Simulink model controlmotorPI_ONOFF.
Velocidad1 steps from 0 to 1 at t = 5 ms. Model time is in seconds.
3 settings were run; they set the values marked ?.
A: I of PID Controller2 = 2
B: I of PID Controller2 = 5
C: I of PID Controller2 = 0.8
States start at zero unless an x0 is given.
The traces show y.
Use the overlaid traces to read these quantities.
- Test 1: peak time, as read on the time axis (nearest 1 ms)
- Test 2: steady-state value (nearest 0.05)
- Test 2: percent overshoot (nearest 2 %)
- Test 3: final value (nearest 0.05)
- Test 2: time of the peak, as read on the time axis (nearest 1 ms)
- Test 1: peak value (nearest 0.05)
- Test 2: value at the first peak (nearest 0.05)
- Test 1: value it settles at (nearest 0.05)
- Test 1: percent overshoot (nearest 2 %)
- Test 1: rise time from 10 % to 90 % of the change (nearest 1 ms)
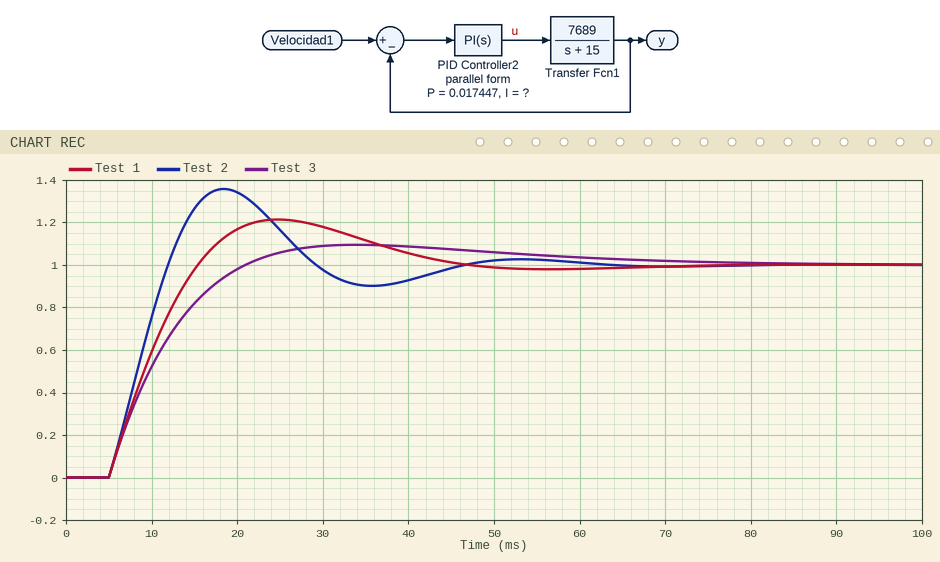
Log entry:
25 ms
1.00
36 %
1.00
18 ms
1.20
1.35
1.00
22 %
8 ms
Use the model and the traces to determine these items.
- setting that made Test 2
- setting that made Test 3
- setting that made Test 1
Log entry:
B
C
A
